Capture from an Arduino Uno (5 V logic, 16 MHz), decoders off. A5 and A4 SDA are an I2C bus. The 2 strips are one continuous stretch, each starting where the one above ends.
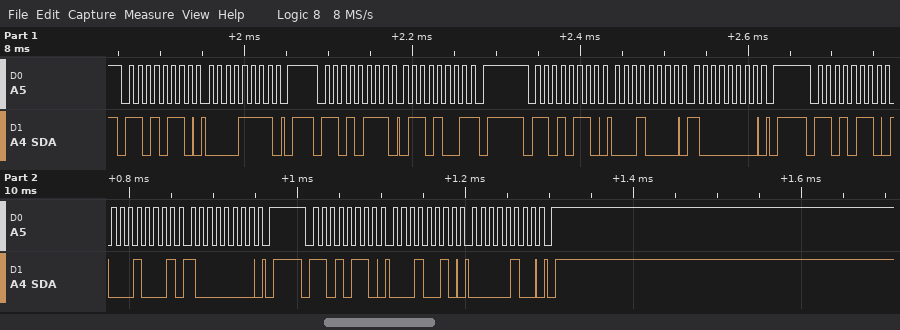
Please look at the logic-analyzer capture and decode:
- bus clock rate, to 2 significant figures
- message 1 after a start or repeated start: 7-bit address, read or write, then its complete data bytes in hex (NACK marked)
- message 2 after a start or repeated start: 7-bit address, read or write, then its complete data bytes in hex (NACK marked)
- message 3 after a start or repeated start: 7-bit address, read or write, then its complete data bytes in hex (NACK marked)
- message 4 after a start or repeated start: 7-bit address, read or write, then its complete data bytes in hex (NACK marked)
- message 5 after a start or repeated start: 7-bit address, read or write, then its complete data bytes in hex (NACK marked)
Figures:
100 kHz
0x6B write: 0F
0x6B read: 69 NACK
0x6B write: 10 80
0x6B write: 11 80
0x6B write: 12 04
